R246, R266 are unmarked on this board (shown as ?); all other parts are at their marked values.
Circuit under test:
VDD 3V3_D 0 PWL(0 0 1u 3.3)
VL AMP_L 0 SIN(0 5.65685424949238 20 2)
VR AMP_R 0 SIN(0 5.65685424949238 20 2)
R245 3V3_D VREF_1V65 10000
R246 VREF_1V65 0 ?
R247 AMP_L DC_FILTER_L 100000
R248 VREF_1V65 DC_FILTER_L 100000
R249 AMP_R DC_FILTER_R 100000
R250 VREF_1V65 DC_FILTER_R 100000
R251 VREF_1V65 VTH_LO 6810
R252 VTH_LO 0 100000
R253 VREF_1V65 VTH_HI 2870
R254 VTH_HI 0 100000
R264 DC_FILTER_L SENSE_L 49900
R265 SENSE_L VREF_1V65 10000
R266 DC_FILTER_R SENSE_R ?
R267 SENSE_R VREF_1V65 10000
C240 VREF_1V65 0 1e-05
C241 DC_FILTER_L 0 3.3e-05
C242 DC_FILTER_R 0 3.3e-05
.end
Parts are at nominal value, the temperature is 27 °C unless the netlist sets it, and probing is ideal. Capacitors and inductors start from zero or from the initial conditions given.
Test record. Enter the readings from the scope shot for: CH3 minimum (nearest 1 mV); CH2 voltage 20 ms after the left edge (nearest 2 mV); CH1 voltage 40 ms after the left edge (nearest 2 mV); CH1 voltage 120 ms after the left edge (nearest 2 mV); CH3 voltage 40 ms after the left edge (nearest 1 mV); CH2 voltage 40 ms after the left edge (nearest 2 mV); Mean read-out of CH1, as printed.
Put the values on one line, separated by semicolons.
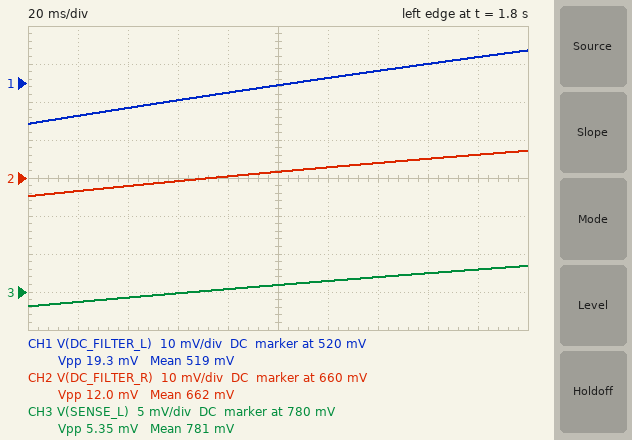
778 mV; 656 mV; 514 mV; 522 mV; 779 mV; 658 mV; 519 mV
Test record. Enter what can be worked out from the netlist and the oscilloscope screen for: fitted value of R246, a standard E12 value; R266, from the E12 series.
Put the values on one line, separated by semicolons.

3.9 kΩ; 15 kΩ
